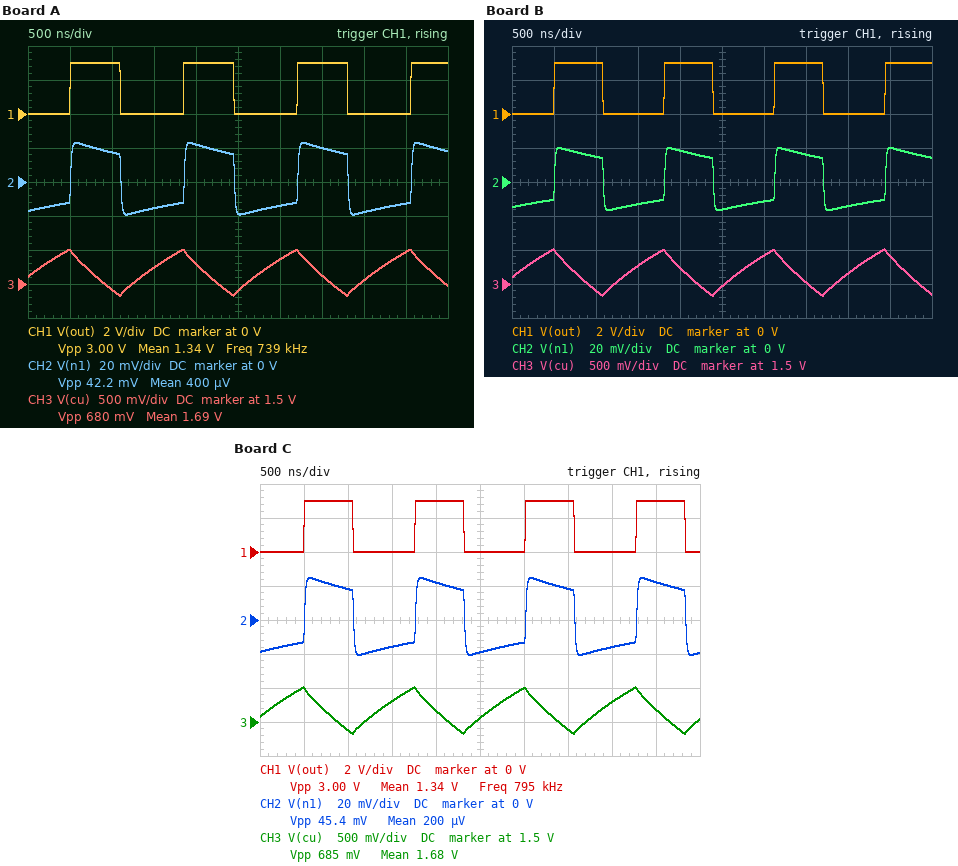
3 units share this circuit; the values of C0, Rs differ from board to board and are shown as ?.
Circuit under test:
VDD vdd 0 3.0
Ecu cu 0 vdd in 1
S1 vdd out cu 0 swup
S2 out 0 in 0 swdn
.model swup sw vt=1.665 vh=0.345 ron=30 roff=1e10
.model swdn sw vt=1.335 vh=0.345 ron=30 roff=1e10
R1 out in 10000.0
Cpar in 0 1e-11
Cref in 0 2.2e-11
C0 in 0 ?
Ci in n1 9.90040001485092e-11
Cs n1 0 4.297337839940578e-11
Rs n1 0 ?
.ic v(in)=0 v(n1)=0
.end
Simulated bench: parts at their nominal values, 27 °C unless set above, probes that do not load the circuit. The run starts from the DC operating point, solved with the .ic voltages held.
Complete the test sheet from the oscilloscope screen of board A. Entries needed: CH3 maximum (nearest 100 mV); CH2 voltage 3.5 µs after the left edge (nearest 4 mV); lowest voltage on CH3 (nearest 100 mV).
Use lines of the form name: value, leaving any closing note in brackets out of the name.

CH3 maximum: 2.0 V
CH2 voltage 3.5 µs after the left edge: 20 mV
lowest voltage on CH3: 1.3 V
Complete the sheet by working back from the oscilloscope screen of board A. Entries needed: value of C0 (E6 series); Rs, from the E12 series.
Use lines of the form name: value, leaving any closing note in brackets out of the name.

value of C0: 15 pF
Rs, from the E12 series: 180 Ω
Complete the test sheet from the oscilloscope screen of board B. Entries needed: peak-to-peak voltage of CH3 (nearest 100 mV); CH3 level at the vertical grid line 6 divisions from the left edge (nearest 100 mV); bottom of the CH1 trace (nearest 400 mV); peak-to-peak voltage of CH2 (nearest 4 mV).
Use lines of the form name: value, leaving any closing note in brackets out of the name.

peak-to-peak voltage of CH3: 700 mV
CH3 level at the vertical grid line 6 divisions from the left edge: 1.9 V
bottom of the CH1 trace: 0 V
peak-to-peak voltage of CH2: 36 mV
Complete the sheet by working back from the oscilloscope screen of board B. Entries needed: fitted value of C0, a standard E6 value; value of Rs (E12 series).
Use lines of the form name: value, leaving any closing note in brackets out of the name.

fitted value of C0, a standard E6 value: 10 pF
value of Rs: 150 Ω
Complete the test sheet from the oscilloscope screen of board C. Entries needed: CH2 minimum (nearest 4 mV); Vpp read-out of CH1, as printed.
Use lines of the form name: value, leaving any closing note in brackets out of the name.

CH2 minimum: -20 mV
Vpp read-out of CH1, as printed: 3.00 V
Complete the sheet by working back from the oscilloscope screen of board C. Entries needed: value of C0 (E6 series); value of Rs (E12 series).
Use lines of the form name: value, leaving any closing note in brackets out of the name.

value of C0: 4.7 pF
value of Rs: 180 Ω
